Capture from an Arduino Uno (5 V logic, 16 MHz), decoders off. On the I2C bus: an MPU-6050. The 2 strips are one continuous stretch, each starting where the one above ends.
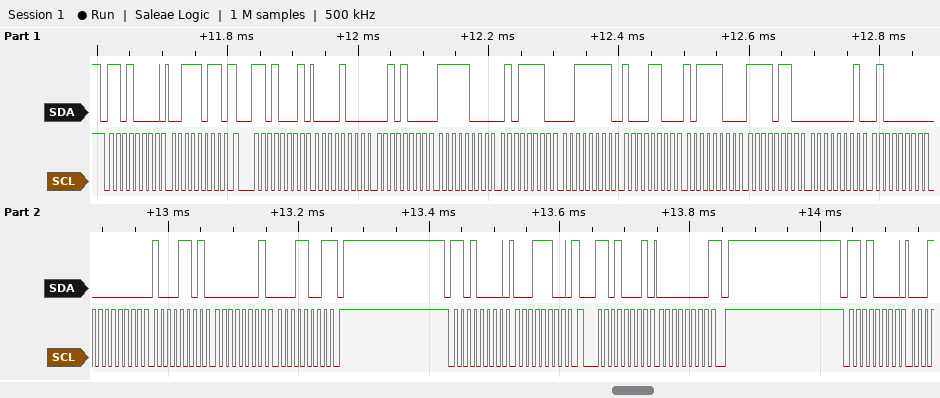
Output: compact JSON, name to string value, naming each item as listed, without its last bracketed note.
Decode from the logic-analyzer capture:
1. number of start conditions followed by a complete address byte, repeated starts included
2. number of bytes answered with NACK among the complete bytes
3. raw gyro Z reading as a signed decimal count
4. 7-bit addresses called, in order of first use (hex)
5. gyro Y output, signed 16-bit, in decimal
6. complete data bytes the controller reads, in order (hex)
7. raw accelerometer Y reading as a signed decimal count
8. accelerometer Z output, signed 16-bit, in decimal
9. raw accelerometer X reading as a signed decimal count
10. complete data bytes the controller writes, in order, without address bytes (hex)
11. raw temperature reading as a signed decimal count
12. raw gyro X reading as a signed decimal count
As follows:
{"number of start conditions followed by a complete address byte, repeated starts included": "5", "number of bytes answered with NACK among the complete bytes": "2", "raw gyro Z reading as a signed decimal count": "281", "7-bit addresses called, in order of first use": "0x68", "gyro Y output, signed 16-bit, in decimal": "141", "complete data bytes the controller reads, in order": "08 28 F8 5E 3F 8C BC F6 01 40 00 8D 01 19 00", "raw accelerometer Y reading as a signed decimal count": "-1954", "accelerometer Z output, signed 16-bit, in decimal": "16268", "raw accelerometer X reading as a signed decimal count": "2088", "complete data bytes the controller writes, in order, without address bytes": "3B 1C", "raw temperature reading as a signed decimal count": "-17162", "raw gyro X reading as a signed decimal count": "320"}
